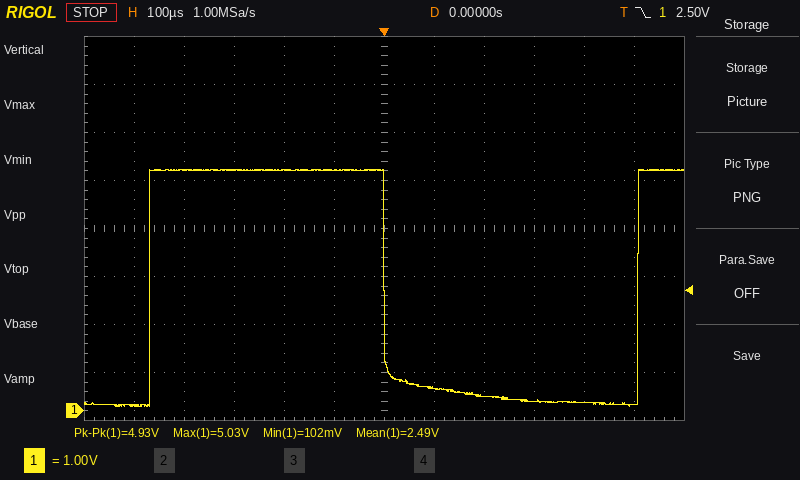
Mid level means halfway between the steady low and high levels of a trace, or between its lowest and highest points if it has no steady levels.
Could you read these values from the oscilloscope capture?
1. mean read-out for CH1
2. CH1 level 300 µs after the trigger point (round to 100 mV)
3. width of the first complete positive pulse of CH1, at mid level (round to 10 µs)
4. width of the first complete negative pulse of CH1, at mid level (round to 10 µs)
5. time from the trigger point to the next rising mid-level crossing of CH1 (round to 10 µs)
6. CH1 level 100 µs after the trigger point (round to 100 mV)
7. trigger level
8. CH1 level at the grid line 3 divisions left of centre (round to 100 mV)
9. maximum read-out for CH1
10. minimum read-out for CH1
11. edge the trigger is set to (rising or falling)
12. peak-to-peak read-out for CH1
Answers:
2.49 V
200 mV
470 µs
510 µs
510 µs
500 mV
2.50 V
5.0 V
5.03 V
102 mV
falling
4.93 V
